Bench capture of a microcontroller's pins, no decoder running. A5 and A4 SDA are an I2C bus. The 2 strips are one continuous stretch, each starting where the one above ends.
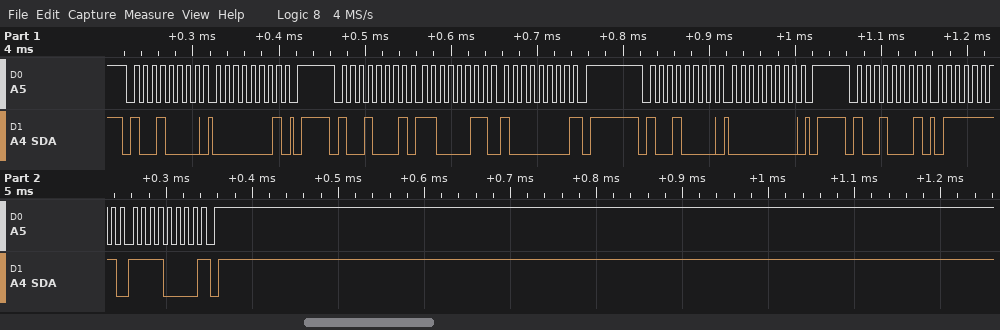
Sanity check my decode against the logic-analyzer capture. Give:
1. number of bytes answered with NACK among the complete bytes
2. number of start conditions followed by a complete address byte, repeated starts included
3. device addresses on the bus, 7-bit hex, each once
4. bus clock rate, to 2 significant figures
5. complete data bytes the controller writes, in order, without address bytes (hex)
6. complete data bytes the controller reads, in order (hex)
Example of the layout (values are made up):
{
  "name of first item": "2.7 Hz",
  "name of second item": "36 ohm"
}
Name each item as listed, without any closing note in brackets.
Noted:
{
  "number of bytes answered with NACK among the complete bytes": "2",
  "number of start conditions followed by a complete address byte, repeated starts included": "4",
  "device addresses on the bus, 7-bit hex, each once": "0x48",
  "bus clock rate, to 2 significant figures": "100 kHz",
  "complete data bytes the controller writes, in order, without address bytes": "01 00",
  "complete data bytes the controller reads, in order": "C3 80 7F F0"
}
